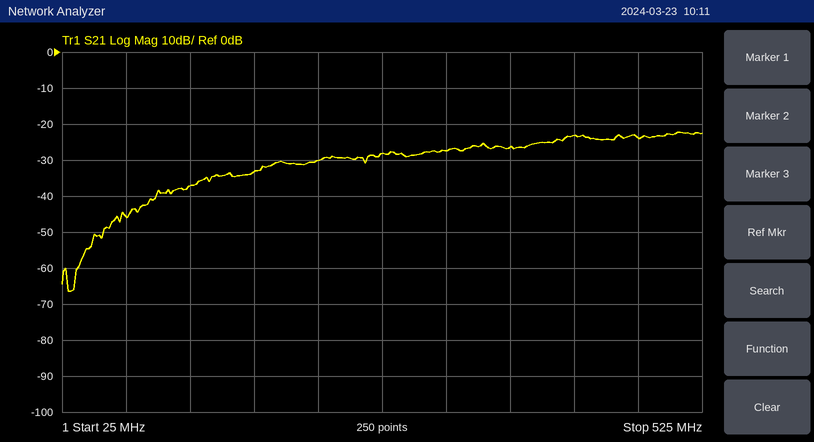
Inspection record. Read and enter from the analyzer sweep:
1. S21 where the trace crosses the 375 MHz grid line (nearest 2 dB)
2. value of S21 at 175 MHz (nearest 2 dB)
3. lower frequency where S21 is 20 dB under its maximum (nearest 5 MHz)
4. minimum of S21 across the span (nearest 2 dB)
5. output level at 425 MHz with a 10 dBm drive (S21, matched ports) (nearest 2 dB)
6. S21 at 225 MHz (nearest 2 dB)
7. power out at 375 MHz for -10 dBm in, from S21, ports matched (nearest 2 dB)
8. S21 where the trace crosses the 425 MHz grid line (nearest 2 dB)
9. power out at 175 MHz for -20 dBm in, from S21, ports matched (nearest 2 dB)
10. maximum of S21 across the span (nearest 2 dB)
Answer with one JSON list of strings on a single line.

["-26 dB", "-34 dB", "90 MHz", "-66 dB", "-14 dBm", "-30 dB", "-36 dBm", "-24 dB", "-54 dBm", "-22 dB"]
